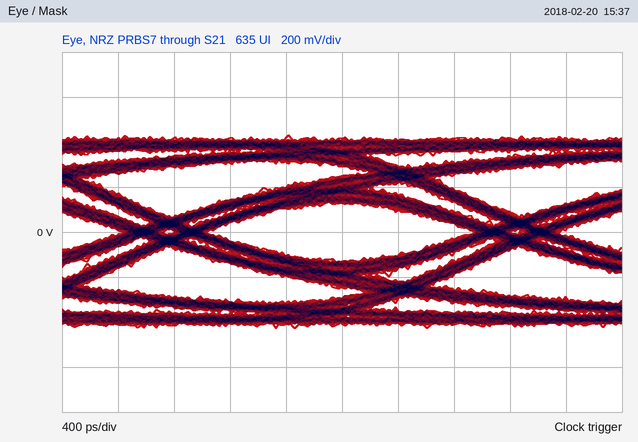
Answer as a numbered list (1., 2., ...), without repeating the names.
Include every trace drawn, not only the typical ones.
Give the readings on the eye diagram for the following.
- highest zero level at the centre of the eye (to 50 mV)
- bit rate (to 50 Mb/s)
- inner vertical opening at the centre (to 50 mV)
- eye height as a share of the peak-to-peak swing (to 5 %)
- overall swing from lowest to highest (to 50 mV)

1. -150 mV
2. 400 Mb/s
3. 250 mV
4. 30 %
5. 850 mV
